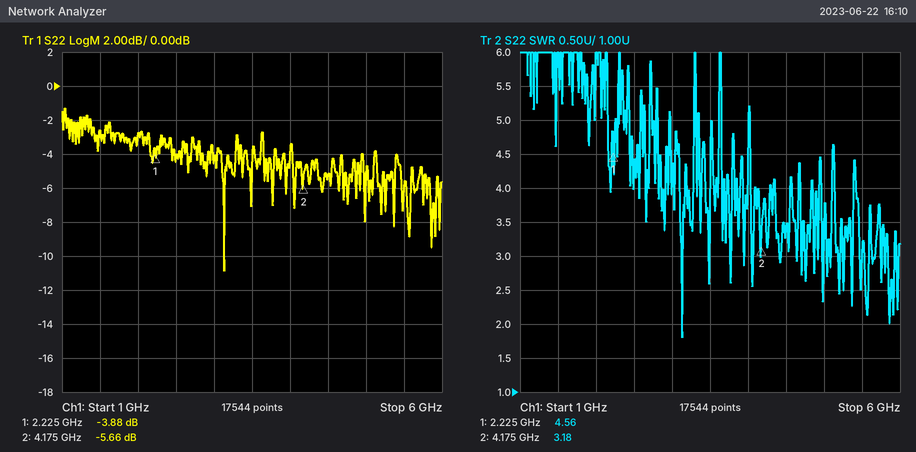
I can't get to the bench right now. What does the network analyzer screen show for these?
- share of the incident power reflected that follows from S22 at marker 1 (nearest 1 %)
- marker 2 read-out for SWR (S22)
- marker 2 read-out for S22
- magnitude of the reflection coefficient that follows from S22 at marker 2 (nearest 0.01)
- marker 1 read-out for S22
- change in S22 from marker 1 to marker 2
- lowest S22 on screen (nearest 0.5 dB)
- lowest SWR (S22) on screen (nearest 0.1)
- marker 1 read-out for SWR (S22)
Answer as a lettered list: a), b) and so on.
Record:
a) 41 %
b) 3.18
c) -5.66 dB
d) 0.52
e) -3.88 dB
f) -1.78 dB
g) -11.0 dB
h) 1.8
i) 4.56
